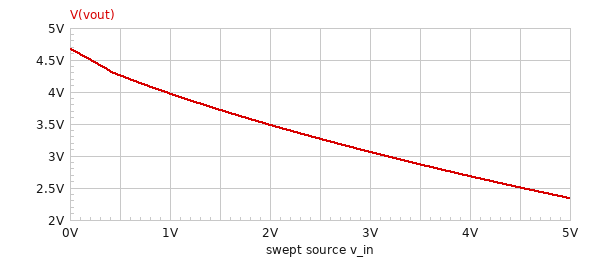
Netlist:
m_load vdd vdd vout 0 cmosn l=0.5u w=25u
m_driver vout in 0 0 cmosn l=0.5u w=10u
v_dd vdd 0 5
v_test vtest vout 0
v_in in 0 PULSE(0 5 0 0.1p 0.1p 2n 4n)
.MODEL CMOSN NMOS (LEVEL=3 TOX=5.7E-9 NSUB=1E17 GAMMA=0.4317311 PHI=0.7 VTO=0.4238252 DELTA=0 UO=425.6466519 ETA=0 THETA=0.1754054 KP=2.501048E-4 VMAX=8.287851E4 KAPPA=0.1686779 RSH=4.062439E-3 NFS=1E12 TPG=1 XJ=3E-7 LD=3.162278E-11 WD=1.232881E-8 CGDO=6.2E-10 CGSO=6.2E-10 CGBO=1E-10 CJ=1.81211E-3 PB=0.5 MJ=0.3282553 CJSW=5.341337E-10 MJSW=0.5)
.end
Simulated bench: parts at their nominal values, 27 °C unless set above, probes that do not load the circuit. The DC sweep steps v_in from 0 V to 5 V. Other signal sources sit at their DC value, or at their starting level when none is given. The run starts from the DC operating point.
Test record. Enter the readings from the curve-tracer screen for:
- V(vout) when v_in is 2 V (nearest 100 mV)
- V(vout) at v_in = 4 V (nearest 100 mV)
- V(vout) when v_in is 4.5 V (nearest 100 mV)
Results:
3.5 V
2.7 V
2.5 V
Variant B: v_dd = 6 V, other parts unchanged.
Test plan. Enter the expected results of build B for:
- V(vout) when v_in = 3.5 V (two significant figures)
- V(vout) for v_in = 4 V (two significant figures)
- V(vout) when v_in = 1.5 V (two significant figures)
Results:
3.8 V
3.6 V
4.7 V
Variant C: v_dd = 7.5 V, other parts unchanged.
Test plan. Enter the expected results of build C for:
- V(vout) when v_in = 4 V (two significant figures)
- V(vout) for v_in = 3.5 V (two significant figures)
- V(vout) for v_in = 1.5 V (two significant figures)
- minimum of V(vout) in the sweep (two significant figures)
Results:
5.0 V
5.2 V
6.1 V
4.6 V
